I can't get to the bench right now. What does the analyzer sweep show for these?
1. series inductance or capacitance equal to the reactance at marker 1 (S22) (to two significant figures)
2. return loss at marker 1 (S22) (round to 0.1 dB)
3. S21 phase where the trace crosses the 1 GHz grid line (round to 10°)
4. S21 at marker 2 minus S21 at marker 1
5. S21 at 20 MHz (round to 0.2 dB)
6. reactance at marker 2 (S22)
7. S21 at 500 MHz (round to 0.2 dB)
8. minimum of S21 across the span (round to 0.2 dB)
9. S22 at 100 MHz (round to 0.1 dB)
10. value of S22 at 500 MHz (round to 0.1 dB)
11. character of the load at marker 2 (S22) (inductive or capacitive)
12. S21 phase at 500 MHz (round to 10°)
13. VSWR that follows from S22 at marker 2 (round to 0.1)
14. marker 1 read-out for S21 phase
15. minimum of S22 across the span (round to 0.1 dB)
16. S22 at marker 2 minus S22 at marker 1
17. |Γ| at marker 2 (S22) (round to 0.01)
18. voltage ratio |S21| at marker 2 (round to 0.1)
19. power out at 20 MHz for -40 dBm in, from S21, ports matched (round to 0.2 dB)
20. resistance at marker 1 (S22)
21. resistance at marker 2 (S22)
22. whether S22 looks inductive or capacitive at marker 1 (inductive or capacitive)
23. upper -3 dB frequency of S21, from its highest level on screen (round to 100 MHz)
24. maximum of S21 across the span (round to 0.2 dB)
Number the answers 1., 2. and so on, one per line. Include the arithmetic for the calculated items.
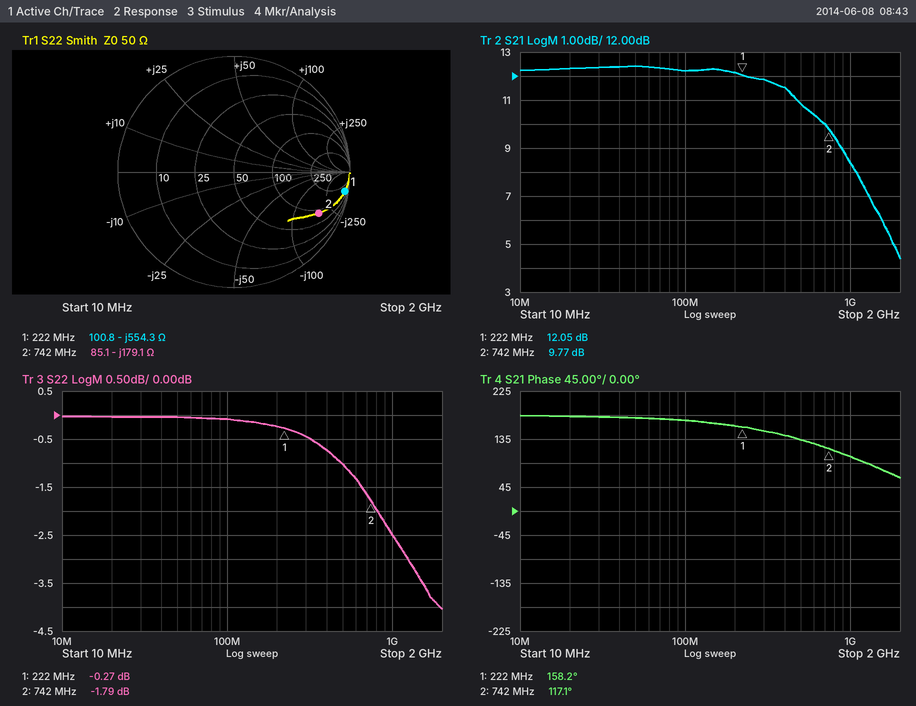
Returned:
1. C = 1/(2π × 222 MHz × 554.3 Ω) ≈ 1.3 pF
2. 0.3 dB
3. 100°
4. 9.77 − (12.05) = -2.28 dB
5. 12.4 dB
6. -179.1 Ω
7. 10.8 dB
8. 4.4 dB
9. -0.1 dB
10. -1.0 dB
11. capacitive
12. 130°
13. (1 + 0.8138)/(1 − 0.8138) ≈ 9.7
14. 158.2°
15. -4.0 dB
16. -1.79 − (-0.27) = -1.52 dB
17. 0.81
18. 10^(9.77/20) ≈ 3.1
19. -40 dBm + (12.4 dB) = -27.6 dBm
20. 100.8 Ω
21. 85.1 Ω
22. capacitive
23. 800 MHz
24. 12.4 dB
